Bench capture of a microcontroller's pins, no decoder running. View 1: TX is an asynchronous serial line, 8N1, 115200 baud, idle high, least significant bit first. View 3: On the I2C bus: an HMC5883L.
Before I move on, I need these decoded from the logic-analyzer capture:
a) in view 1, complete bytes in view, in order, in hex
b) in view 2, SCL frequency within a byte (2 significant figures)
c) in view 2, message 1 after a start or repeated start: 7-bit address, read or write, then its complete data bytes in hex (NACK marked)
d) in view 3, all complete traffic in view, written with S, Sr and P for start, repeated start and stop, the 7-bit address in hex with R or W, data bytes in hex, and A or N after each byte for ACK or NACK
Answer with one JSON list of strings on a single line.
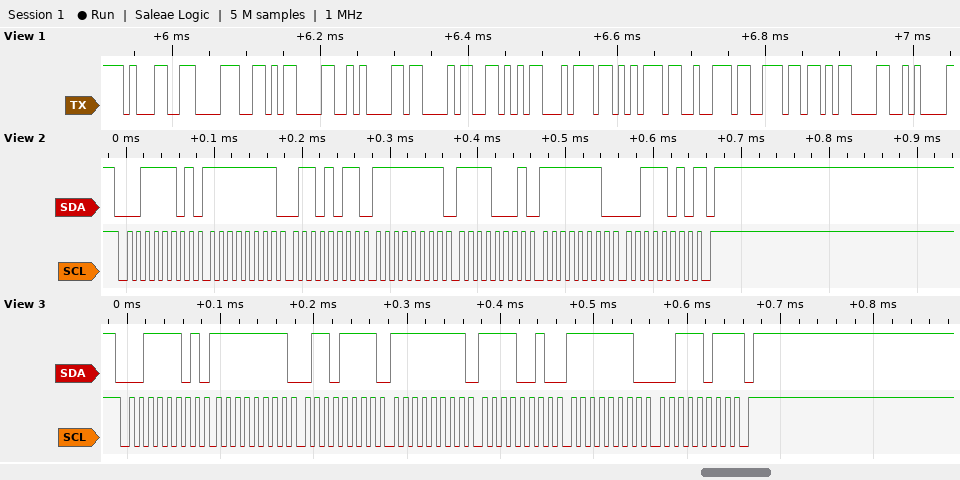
["31 38 0D 0A 43 56 74 75 72 6E 0D 0A", "100 kHz", "0x1E read: FF 6B FF F1 FE 3A NACK", "S 1ER A FF A 6F A FF A F2 A FE A 3B N P"]
